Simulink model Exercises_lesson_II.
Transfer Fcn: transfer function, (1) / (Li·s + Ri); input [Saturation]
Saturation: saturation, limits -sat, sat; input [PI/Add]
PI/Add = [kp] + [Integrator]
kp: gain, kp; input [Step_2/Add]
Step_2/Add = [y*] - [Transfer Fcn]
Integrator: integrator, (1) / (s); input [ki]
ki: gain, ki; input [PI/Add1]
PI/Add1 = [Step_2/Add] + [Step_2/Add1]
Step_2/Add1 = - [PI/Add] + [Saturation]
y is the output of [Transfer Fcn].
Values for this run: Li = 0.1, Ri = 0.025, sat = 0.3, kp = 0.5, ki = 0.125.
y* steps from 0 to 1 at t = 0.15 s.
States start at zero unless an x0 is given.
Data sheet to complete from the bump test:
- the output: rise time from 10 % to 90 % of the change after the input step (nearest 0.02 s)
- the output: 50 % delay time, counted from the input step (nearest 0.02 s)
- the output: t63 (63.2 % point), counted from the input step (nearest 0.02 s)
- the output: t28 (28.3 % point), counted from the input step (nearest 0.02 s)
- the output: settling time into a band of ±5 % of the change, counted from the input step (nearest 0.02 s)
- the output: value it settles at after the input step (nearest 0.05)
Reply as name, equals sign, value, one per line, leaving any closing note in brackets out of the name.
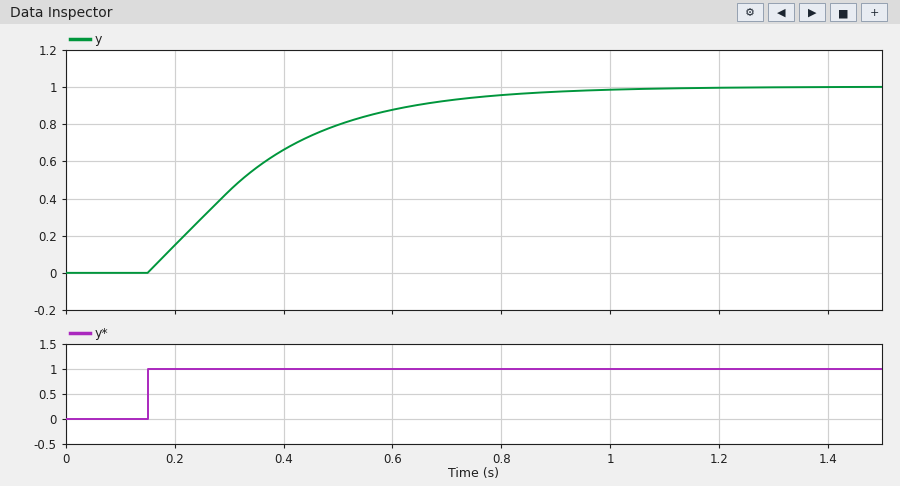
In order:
the output: rise time from 10 % to 90 % of the change after the input step = 0.46 s
the output: 50 % delay time, counted from the input step = 0.18 s
the output: t63 (63.2 % point), counted from the input step = 0.24 s
the output: t28 (28.3 % point), counted from the input step = 0.10 s
the output: settling time into a band of ±5 % of the change, counted from the input step = 0.62 s
the output: value it settles at after the input step = 1.00
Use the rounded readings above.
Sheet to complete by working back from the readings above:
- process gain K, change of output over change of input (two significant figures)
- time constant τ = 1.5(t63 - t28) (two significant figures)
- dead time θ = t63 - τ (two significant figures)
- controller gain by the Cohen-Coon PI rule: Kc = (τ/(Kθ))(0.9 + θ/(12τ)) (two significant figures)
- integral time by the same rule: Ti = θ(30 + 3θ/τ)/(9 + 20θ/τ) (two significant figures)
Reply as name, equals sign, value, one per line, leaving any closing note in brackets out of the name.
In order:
process gain K, change of output over change of input = 1.0
time constant τ = 1.5(t63 - t28) = 0.21 s
dead time θ = t63 - τ = 0.030 s
controller gain by the Cohen-Coon PI rule: Kc = (τ/(Kθ))(0.9 + θ/(12τ)) = 6.4
integral time by the same rule: Ti = θ(30 + 3θ/τ)/(9 + 20θ/τ) = 0.077 s
